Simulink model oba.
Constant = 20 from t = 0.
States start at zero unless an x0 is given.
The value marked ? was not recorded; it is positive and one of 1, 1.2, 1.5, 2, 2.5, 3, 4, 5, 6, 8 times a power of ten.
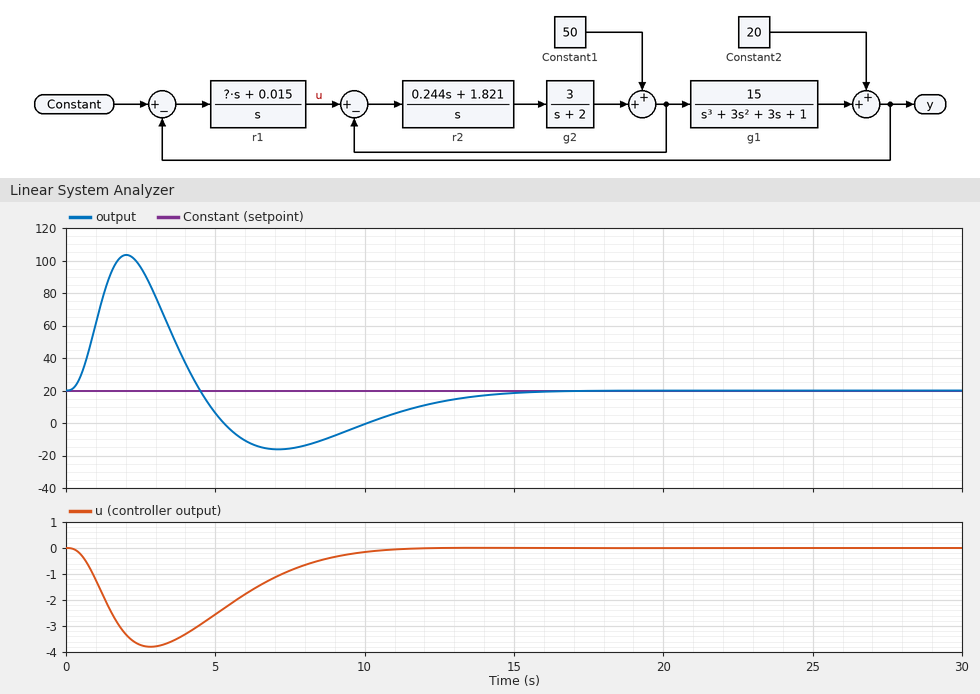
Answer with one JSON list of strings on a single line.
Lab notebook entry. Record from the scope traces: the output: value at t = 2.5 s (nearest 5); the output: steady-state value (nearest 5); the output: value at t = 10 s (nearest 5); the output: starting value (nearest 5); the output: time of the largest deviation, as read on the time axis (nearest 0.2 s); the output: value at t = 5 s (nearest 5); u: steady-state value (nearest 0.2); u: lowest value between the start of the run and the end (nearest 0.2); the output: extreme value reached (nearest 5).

["95", "20", "0", "20", "2.0 s", "5", "0.0", "-3.8", "105"]
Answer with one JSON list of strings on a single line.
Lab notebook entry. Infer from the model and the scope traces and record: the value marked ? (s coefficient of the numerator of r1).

["0.025"]
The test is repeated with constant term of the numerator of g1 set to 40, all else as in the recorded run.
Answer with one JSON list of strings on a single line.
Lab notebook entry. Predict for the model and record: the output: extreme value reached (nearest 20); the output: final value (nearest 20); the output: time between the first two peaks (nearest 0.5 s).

["240", "20", "8.5 s"]
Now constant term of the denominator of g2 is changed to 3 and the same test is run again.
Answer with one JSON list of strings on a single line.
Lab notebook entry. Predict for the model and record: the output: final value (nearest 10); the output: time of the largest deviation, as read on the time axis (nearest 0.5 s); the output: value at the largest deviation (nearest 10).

["20", "2.5 s", "130"]
